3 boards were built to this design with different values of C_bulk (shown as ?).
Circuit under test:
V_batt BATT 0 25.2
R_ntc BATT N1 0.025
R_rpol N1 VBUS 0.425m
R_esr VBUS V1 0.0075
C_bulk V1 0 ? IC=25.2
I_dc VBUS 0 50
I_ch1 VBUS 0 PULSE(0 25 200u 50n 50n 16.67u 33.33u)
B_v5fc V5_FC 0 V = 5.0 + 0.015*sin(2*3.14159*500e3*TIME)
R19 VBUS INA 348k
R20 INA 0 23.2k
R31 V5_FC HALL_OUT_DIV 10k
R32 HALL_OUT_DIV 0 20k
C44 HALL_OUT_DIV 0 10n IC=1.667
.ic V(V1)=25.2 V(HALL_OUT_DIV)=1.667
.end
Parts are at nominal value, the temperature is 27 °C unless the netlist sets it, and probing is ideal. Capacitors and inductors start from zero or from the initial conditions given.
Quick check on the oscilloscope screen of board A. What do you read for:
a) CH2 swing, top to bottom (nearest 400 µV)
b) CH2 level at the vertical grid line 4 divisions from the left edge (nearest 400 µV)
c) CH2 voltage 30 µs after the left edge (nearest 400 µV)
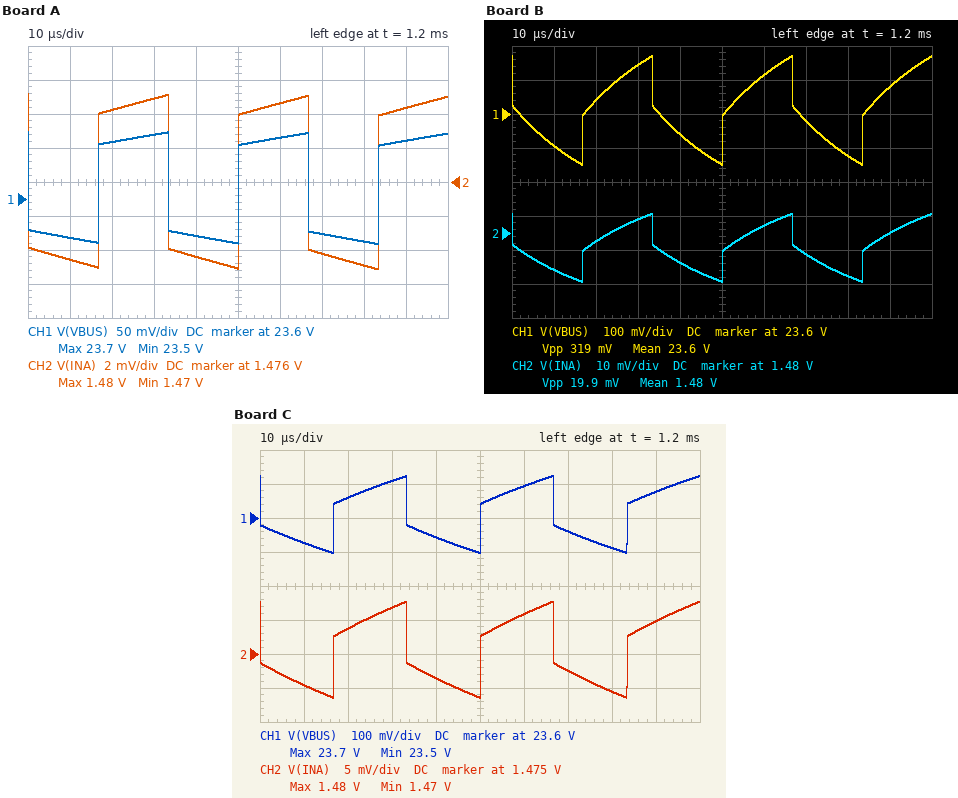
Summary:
10.4 mV
1.4716 V
1.4808 V
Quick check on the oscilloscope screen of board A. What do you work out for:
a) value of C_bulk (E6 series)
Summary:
6.8 mF
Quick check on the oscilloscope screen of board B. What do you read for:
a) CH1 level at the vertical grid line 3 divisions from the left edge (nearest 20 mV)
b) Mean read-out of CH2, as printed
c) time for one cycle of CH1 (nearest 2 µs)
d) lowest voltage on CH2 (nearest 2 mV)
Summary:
23.74 V
1.48 V
34 µs
1.466 V
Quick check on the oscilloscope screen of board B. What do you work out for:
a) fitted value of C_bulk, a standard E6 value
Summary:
680 µF
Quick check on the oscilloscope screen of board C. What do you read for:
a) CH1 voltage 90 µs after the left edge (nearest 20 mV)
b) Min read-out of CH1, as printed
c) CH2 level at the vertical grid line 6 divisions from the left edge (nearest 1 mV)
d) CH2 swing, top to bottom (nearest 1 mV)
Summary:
23.68 V
23.5 V
1.481 V
14 mV
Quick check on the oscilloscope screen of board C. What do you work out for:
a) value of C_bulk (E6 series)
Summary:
1.5 mF
